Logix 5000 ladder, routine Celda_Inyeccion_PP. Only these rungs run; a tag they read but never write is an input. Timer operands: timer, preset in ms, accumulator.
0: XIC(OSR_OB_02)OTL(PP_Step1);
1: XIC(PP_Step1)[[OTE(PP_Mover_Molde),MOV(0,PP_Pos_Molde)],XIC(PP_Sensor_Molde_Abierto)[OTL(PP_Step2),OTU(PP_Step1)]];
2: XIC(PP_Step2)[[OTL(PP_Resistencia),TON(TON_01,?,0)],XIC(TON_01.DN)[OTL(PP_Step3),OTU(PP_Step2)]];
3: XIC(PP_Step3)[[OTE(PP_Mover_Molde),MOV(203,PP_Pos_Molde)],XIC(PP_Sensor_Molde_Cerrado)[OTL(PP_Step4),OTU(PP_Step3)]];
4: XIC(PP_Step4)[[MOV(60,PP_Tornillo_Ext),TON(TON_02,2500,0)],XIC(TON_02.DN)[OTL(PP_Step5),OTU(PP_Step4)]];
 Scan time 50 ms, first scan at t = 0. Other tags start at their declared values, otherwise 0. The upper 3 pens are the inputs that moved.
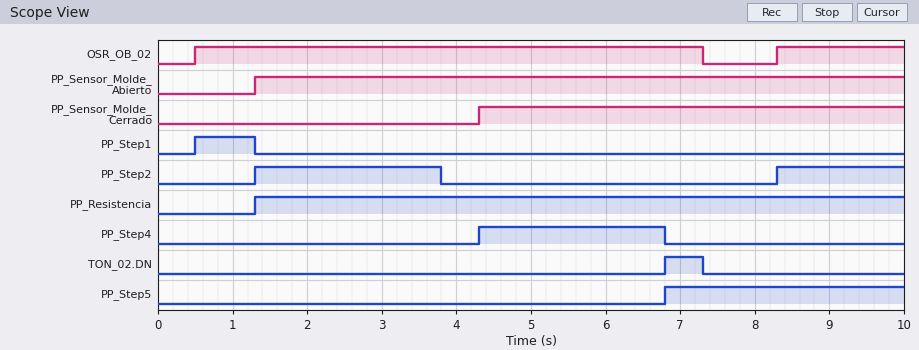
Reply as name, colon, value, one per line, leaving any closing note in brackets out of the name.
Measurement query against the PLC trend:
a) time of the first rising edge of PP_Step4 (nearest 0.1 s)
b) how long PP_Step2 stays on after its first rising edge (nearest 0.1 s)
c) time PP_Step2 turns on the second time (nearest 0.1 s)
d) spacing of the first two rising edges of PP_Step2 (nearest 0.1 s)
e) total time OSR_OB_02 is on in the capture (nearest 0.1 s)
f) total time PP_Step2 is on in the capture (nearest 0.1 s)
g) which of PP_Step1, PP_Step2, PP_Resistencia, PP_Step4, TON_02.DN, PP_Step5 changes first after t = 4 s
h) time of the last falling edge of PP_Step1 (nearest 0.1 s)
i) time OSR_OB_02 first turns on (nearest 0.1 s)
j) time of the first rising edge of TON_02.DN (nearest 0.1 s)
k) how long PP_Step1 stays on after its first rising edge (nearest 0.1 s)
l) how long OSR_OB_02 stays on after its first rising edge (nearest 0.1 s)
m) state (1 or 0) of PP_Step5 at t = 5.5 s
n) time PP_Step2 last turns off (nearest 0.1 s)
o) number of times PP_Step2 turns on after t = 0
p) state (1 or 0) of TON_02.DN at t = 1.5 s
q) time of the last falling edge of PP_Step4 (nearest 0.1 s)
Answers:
time of the first rising edge of PP_Step4: 4.3 s
how long PP_Step2 stays on after its first rising edge: 2.5 s
time PP_Step2 turns on the second time: 8.3 s
spacing of the first two rising edges of PP_Step2: 7.0 s
total time OSR_OB_02 is on in the capture: 8.5 s
total time PP_Step2 is on in the capture: 4.2 s
which of PP_Step1, PP_Step2, PP_Resistencia, PP_Step4, TON_02.DN, PP_Step5 changes first after t = 4 s: PP_Step4
time of the last falling edge of PP_Step1: 1.3 s
time OSR_OB_02 first turns on: 0.5 s
time of the first rising edge of TON_02.DN: 6.8 s
how long PP_Step1 stays on after its first rising edge: 0.8 s
how long OSR_OB_02 stays on after its first rising edge: 6.8 s
state (1 or 0) of PP_Step5 at t = 5.5 s: 0
time PP_Step2 last turns off: 3.8 s
number of times PP_Step2 turns on after t = 0: 2
state (1 or 0) of TON_02.DN at t = 1.5 s: 0
time of the last falling edge of PP_Step4: 6.8 s
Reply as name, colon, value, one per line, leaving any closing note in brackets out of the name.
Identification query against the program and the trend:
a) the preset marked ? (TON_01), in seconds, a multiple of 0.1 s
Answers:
the preset marked ? (TON_01), in seconds, a multiple of 0.1 s: 2.5 s
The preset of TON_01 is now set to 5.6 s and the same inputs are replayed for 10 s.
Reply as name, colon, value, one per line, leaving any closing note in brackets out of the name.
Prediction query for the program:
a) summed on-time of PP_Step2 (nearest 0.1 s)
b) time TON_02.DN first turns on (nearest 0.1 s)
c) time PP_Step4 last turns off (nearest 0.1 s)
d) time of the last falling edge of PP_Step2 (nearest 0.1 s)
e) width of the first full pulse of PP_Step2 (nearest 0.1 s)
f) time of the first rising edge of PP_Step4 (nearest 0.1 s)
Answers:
summed on-time of PP_Step2: 7.3 s
time TON_02.DN first turns on: 9.4 s
time PP_Step4 last turns off: 9.4 s
time of the last falling edge of PP_Step2: 6.9 s
width of the first full pulse of PP_Step2: 5.6 s
time of the first rising edge of PP_Step4: 6.9 s
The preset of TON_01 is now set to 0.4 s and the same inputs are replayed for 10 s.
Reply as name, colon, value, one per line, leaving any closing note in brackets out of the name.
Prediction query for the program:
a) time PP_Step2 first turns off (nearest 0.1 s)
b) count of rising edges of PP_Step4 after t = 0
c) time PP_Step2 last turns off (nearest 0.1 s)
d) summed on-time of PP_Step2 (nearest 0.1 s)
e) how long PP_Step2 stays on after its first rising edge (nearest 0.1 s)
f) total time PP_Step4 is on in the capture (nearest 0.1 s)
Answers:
time PP_Step2 first turns off: 1.7 s
count of rising edges of PP_Step4 after t = 0: 2
time PP_Step2 last turns off: 8.7 s
summed on-time of PP_Step2: 0.8 s
how long PP_Step2 stays on after its first rising edge: 0.4 s
total time PP_Step4 is on in the capture: 3.8 s
